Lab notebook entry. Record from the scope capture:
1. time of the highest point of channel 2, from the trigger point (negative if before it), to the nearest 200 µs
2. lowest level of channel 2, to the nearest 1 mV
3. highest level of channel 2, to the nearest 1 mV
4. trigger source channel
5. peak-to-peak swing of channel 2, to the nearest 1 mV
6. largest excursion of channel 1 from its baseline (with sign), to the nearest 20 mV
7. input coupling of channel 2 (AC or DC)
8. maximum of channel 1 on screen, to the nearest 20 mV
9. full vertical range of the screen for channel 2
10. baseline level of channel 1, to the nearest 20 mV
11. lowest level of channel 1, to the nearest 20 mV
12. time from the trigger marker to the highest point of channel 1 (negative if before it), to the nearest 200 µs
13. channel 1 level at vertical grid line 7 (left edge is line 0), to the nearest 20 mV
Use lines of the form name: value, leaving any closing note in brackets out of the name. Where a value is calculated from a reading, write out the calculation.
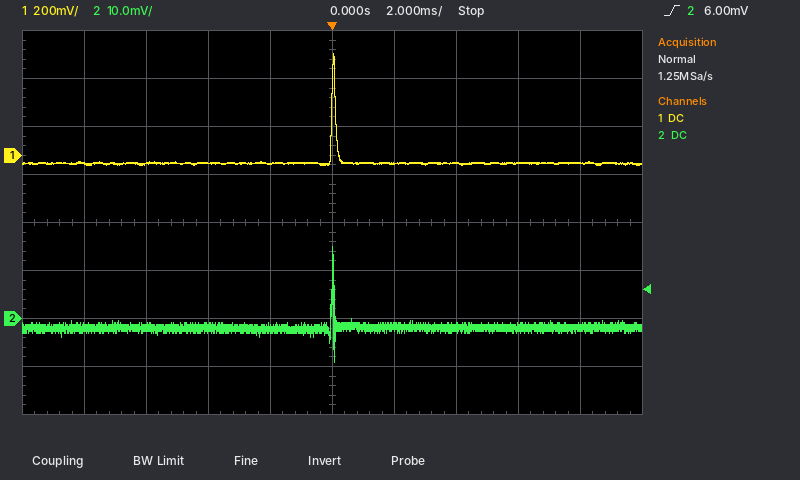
time of the highest point of channel 2, from the trigger point (negative if before it), to the nearest 200 µs: 0.0 ms
lowest level of channel 2, to the nearest 1 mV: -9 mV
highest level of channel 2, to the nearest 1 mV: 15 mV
trigger source channel: channel 2
peak-to-peak swing of channel 2, to the nearest 1 mV: 15 mV − (-9 mV) = 24 mV
largest excursion of channel 1 from its baseline (with sign), to the nearest 20 mV: 420 mV − (-40 mV) = +460 mV
input coupling of channel 2: DC
maximum of channel 1 on screen, to the nearest 20 mV: 420 mV
full vertical range of the screen for channel 2: 80 mV
baseline level of channel 1, to the nearest 20 mV: -40 mV
lowest level of channel 1, to the nearest 20 mV: -40 mV
time from the trigger marker to the highest point of channel 1 (negative if before it), to the nearest 200 µs: 0.0 ms
channel 1 level at vertical grid line 7 (left edge is line 0), to the nearest 20 mV: -40 mV
